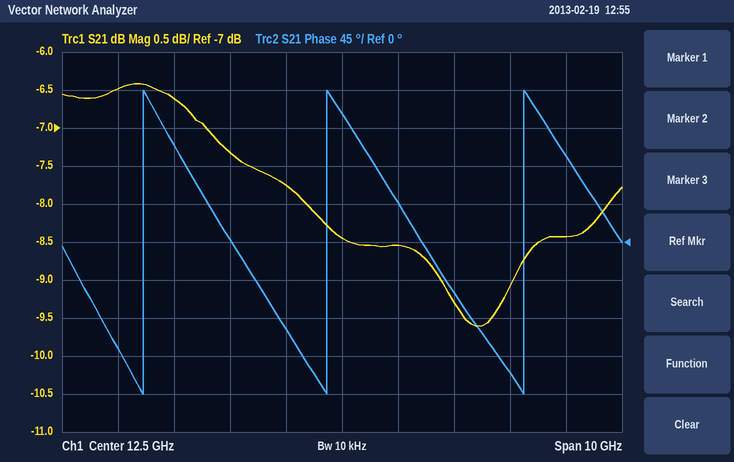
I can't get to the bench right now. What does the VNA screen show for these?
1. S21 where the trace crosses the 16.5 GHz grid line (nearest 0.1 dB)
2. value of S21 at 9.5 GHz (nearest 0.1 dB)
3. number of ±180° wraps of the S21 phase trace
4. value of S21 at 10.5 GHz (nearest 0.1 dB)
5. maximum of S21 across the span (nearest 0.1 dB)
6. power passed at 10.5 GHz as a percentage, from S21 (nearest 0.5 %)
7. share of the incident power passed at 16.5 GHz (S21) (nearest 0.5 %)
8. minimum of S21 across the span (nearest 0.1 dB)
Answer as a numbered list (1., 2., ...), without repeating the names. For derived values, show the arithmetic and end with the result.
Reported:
1. -8.4 dB
2. -6.6 dB
3. 3
4. -7.3 dB
5. -6.4 dB
6. 10^(-7.3/10) ≈ 18.6 %, so 18.5 % to the nearest 0.5 %
7. 10^(-8.4/10) ≈ 14.5 %
8. -9.6 dB
